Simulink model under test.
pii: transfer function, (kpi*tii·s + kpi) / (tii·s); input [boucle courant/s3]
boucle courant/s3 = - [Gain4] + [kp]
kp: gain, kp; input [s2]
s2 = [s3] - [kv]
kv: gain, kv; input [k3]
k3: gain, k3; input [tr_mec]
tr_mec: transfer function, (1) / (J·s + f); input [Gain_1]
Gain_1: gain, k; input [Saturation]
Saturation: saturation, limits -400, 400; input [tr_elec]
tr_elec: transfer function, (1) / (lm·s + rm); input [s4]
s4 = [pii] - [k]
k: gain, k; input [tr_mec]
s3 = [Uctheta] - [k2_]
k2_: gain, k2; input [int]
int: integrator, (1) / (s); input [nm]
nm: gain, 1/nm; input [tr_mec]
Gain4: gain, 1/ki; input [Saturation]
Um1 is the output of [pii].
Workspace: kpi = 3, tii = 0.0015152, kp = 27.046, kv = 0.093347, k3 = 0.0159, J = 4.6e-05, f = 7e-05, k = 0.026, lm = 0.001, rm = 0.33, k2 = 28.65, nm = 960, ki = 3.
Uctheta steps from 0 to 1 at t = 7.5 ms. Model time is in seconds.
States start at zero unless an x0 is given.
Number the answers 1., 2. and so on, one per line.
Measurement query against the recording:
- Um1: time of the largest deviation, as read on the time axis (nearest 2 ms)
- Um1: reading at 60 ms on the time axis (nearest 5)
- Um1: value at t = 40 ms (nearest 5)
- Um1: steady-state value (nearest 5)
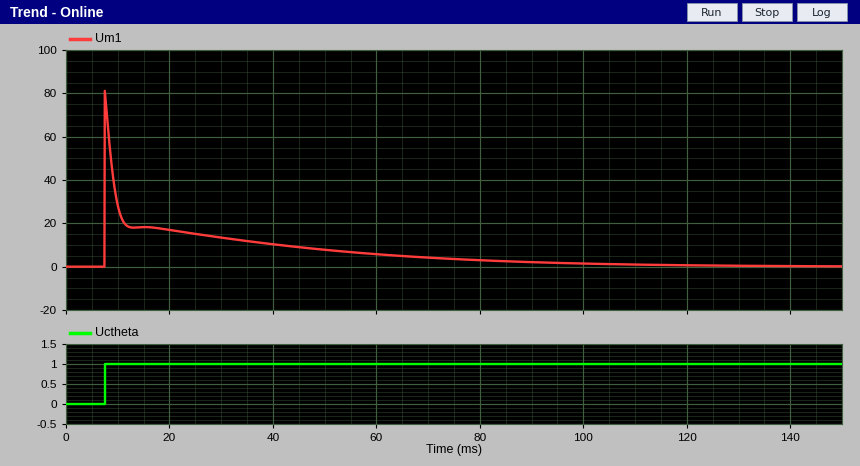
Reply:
1. 8 ms
2. 5
3. 10
4. 0
